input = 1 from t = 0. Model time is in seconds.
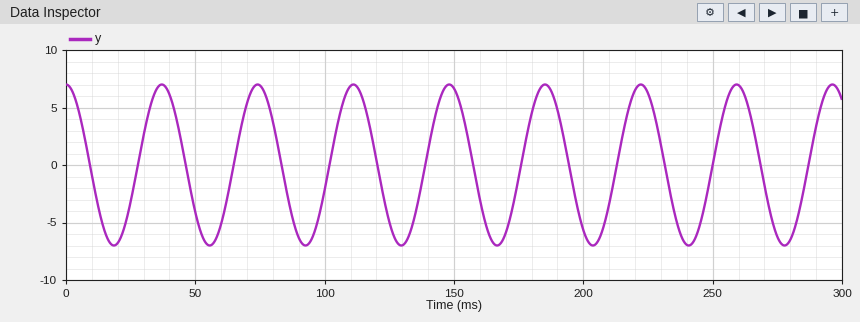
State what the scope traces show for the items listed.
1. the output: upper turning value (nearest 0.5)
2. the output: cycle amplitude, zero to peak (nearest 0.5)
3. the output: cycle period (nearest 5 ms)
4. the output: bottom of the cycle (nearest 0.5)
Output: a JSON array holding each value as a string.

["7.0", "7.0", "35 ms", "-7.0"]
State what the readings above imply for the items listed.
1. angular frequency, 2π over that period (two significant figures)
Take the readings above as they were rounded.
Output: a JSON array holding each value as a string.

["0.18 rad/ms"]
